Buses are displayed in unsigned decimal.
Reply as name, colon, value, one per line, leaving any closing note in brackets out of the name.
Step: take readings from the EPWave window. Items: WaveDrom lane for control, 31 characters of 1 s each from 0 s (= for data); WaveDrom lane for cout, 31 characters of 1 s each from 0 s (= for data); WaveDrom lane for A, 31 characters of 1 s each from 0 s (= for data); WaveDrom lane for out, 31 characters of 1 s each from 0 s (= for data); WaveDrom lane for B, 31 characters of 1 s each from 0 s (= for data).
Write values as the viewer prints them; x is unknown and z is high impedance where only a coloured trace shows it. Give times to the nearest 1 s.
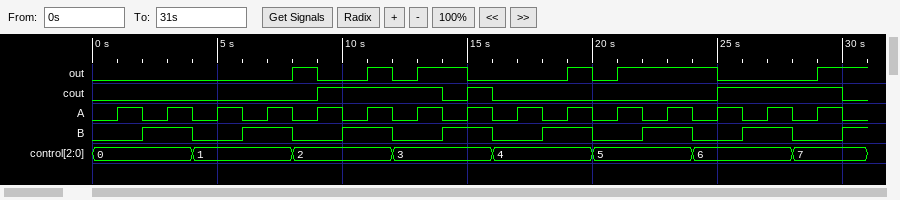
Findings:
WaveDrom lane for control, 31 characters of 1 s each from 0 s: {name: 'control', wave: '=...=...=...=...=...=...=...=..', data: '0 1 2 3 4 5 6 7'}
WaveDrom lane for cout, 31 characters of 1 s each from 0 s: {name: 'cout', wave: '0........1....010........1....0'}
WaveDrom lane for A, 31 characters of 1 s each from 0 s: {name: 'A', wave: '0101010101010101010101010101010'}
WaveDrom lane for out, 31 characters of 1 s each from 0 s: {name: 'out', wave: '0.......10.101.0...101...0...1.'}
WaveDrom lane for B, 31 characters of 1 s each from 0 s: {name: 'B', wave: '0.1.0.1.0.1.0.1.0.1.0.1.0.1.0.1'}
